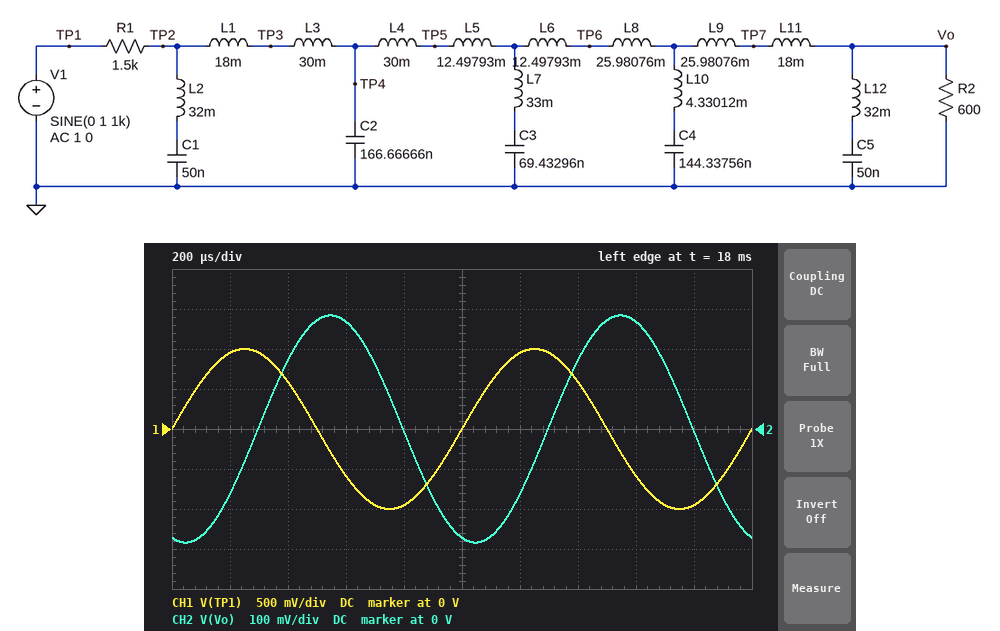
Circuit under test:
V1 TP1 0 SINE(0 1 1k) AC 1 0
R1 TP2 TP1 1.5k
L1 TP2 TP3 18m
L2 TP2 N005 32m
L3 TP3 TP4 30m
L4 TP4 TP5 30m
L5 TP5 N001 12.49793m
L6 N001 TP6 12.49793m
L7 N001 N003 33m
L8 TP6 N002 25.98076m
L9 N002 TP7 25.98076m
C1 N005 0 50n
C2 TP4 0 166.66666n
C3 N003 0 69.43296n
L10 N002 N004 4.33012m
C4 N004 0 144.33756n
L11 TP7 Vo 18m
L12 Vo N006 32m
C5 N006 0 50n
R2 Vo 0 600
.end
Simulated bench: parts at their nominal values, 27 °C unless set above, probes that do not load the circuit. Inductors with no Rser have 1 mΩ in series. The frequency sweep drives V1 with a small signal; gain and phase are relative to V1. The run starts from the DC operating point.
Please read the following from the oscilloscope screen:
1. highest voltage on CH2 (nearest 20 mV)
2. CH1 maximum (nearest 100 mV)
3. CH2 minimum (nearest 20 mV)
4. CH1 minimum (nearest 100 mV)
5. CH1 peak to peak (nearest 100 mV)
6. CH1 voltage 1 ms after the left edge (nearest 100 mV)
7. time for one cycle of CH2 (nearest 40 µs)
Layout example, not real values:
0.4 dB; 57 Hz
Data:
280 mV; 1.0 V; -280 mV; -1.0 V; 2.0 V; 0 V; 1.00 ms
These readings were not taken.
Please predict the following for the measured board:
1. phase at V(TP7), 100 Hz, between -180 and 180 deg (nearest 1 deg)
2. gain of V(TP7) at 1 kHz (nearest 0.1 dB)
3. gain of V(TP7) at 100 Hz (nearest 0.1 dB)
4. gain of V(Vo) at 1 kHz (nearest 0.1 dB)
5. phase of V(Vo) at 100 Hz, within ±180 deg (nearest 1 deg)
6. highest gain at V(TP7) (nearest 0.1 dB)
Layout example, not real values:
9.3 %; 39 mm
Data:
-9 deg; -11.1 dB; -10.9 dB; -10.9 dB; -10 deg; -10.9 dB
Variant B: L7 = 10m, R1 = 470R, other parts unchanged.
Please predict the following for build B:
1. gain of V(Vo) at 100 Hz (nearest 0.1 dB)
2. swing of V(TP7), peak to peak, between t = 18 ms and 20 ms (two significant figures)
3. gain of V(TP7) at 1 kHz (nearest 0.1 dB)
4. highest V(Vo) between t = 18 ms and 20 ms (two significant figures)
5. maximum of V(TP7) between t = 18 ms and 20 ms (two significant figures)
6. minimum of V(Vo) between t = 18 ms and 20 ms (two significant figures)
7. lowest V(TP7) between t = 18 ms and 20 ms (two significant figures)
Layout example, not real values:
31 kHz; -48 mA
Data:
-5.0 dB; 1.1 V; -5.2 dB; 560 mV; 550 mV; -560 mV; -550 mV
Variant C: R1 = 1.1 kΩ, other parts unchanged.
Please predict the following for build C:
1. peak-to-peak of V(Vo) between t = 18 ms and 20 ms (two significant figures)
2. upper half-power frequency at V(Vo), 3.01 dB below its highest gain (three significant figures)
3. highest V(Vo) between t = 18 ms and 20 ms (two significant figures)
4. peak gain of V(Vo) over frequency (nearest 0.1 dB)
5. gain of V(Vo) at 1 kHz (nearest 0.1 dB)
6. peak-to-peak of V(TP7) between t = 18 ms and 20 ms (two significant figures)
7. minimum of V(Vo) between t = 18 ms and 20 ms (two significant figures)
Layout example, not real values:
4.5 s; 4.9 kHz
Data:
700 mV; 3.08 kHz; 350 mV; -9.0 dB; -9.1 dB; 690 mV; -350 mV
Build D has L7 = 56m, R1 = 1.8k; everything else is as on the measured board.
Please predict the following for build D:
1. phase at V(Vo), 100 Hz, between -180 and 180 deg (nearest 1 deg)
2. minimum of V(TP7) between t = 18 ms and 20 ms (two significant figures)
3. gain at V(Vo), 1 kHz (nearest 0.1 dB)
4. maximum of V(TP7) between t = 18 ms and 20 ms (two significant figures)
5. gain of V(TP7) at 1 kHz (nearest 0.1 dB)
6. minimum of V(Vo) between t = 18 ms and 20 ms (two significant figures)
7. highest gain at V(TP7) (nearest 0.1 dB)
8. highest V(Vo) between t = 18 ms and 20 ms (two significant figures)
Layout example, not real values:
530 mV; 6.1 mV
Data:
-10 deg; -240 mV; -12.1 dB; 240 mV; -12.3 dB; -250 mV; -12.0 dB; 250 mV
